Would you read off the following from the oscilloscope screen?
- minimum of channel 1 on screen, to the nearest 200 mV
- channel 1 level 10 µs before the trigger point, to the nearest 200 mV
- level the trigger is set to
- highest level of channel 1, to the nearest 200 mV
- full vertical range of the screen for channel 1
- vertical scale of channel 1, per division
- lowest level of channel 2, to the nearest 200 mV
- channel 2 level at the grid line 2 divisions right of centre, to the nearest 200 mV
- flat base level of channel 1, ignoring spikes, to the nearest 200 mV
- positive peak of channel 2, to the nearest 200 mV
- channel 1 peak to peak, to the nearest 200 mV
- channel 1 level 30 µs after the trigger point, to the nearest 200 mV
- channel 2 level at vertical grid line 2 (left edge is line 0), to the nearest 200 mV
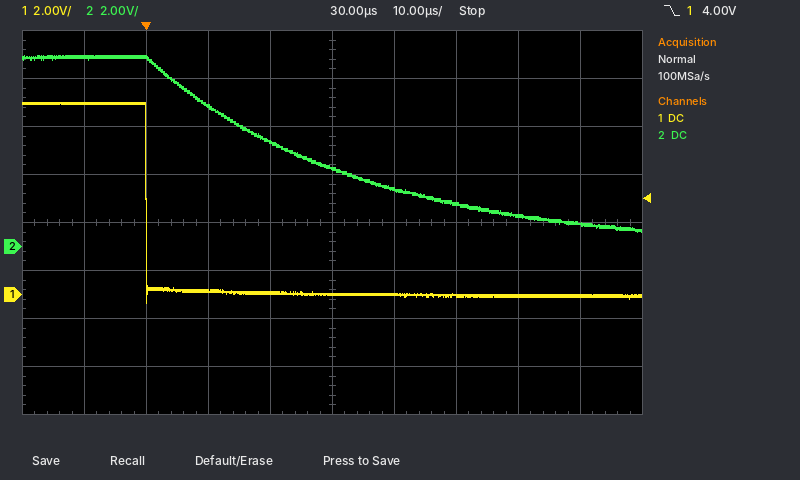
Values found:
-400 mV
8.0 V
4.00 V
8.0 V
16 V
2 V
600 mV
1.8 V
0.0 V
8.0 V
8.4 V
0.0 V
7.8 V
